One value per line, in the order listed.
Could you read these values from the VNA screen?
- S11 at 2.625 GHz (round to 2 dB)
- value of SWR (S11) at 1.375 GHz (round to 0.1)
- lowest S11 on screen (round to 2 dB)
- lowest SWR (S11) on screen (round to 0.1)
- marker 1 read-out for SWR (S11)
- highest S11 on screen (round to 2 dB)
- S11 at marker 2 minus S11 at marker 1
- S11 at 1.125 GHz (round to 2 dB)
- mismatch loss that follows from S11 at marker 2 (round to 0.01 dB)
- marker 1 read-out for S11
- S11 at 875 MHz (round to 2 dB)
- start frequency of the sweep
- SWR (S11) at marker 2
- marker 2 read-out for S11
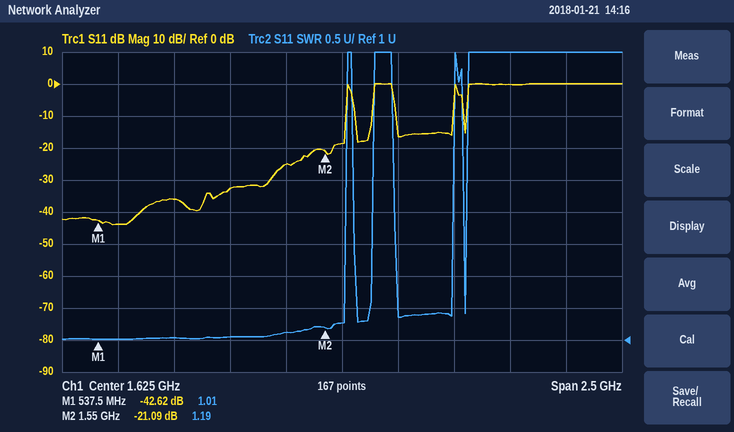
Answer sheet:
0 dB
1.1
-44 dB
1.0
1.01
0 dB
21.53 dB
-32 dB
0.03 dB
-42.62 dB
-36 dB
375 MHz
1.19
-21.09 dB
